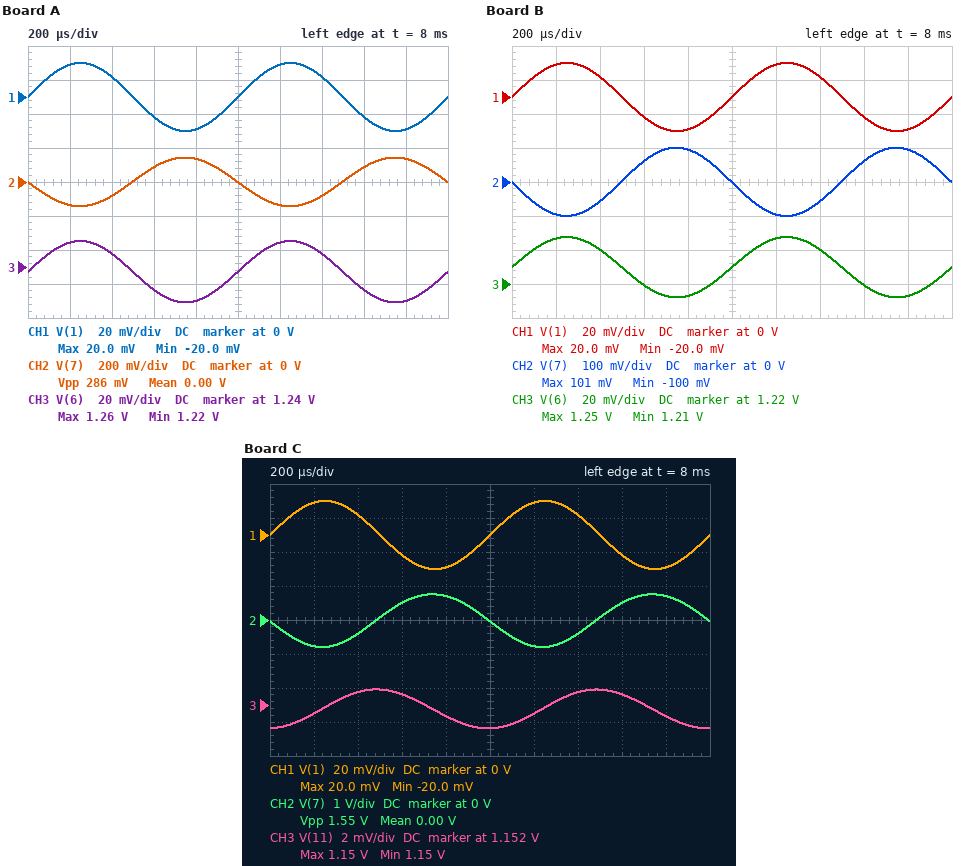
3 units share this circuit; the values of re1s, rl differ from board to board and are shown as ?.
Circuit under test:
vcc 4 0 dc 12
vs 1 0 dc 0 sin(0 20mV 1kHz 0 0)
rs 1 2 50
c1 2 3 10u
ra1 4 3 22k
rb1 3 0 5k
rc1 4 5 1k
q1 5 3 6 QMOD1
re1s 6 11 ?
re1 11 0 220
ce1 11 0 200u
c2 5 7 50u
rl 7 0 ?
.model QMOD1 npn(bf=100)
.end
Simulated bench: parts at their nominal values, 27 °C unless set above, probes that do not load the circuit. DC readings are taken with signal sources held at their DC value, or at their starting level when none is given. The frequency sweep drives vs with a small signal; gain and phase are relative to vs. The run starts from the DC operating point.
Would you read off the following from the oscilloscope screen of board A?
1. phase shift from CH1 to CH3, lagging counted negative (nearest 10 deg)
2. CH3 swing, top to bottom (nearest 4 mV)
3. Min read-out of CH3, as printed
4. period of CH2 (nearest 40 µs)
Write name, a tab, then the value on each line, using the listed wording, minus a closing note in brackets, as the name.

phase shift from CH1 to CH3, lagging counted negative	0 deg
CH3 swing, top to bottom	36 mV
Min read-out of CH3, as printed	1.22 V
period of CH2	1.00 ms
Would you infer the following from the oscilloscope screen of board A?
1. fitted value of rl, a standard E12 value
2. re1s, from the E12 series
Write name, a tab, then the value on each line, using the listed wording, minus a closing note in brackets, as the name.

fitted value of rl, a standard E12 value	1.2 kΩ
re1s, from the E12 series	68 Ω
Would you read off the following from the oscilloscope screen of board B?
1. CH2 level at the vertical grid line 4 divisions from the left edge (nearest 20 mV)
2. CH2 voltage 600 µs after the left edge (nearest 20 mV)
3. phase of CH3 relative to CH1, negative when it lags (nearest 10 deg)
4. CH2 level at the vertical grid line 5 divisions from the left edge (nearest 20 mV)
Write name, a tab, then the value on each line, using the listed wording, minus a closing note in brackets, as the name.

CH2 level at the vertical grid line 4 divisions from the left edge	100 mV
CH2 voltage 600 µs after the left edge	60 mV
phase of CH3 relative to CH1, negative when it lags	0 deg
CH2 level at the vertical grid line 5 divisions from the left edge	0 V
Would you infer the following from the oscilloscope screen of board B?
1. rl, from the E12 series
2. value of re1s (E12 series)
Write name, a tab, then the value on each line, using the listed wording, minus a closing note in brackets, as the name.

rl, from the E12 series	470 Ω
value of re1s	56 Ω
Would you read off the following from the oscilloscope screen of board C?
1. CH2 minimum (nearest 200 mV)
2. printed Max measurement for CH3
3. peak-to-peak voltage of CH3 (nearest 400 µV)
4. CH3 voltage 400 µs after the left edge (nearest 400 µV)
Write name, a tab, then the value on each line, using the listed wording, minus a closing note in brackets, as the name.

CH2 minimum	-800 mV
printed Max measurement for CH3	1.15 V
peak-to-peak voltage of CH3	2.4 mV
CH3 voltage 400 µs after the left edge	1.1528 V
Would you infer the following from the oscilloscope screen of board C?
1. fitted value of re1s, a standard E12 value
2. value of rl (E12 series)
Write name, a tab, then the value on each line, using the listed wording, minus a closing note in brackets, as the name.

fitted value of re1s, a standard E12 value	8.2 Ω
value of rl	1.2 kΩ
